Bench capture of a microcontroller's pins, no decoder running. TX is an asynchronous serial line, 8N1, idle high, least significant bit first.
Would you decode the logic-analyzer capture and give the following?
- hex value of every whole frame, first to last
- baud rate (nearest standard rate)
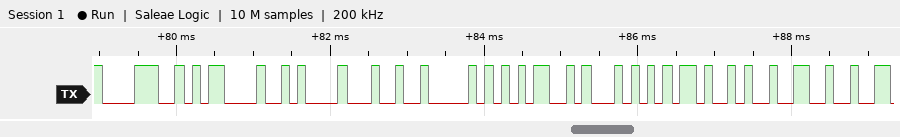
0x38 0x0D 0x0A 0x24 0x50 0x4D 0x54 0x4B 0x32
9600 baud
